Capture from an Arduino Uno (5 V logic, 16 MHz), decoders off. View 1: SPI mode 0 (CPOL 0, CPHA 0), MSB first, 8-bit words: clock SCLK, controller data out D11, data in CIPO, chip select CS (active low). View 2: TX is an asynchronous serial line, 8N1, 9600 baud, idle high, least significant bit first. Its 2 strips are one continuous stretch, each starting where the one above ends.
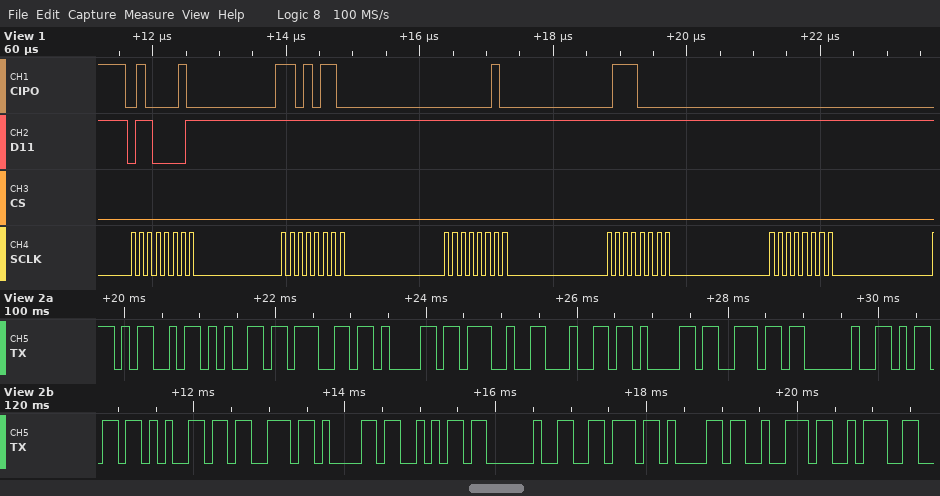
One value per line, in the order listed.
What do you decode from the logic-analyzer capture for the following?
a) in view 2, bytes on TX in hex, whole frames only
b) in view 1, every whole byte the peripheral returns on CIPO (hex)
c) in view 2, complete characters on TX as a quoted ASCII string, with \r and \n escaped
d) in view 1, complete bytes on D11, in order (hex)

4D 65 67 61 27 64 61 6E 20 6D 65 73 61 6A 20 76 61 72 3A
42 D6 02 70 00
"Mega'dan mesaj var:"
61 FF FF FF FF
